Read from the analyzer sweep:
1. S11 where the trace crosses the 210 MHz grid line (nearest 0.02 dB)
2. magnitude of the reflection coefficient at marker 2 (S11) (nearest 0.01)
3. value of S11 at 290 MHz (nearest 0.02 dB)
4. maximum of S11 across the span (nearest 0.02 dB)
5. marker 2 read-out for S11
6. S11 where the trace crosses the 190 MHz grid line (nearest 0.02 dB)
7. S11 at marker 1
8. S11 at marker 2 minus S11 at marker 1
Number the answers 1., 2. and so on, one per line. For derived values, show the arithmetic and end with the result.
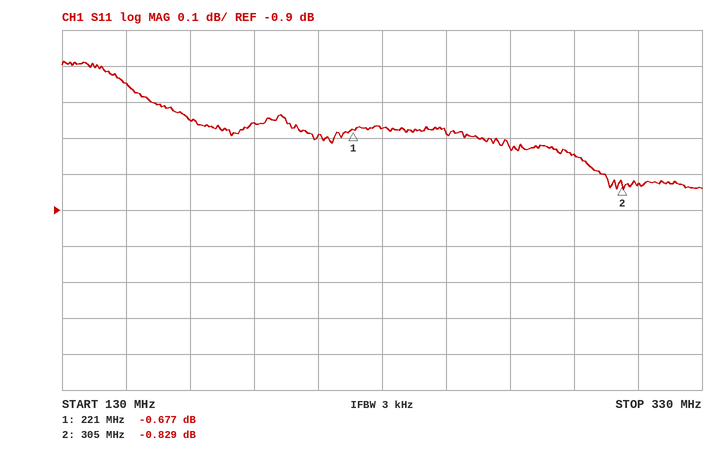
1. -0.70 dB
2. 10^(-0.829/20) ≈ 0.91
3. -0.74 dB
4. -0.48 dB
5. -0.829 dB
6. -0.66 dB
7. -0.677 dB
8. -0.829 − (-0.677) = -0.152 dB
